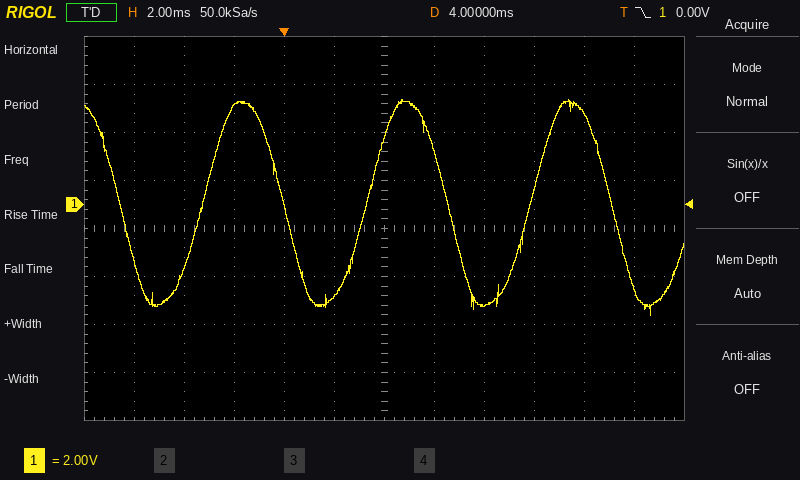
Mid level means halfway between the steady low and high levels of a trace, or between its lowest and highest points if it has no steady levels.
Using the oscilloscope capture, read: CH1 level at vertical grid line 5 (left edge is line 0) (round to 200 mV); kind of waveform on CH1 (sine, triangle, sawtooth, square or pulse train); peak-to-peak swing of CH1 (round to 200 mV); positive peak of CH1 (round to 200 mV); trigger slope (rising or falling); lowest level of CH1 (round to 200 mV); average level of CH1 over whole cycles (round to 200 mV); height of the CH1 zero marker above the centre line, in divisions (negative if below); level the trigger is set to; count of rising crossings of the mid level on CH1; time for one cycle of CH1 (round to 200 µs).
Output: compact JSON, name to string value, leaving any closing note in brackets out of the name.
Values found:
{"CH1 level at vertical grid line 5 (left edge is line 0)": "-3.8 V", "kind of waveform on CH1": "sine", "peak-to-peak swing of CH1": "9.0 V", "positive peak of CH1": "4.4 V", "trigger slope": "falling", "lowest level of CH1": "-4.6 V", "average level of CH1 over whole cycles": "0.0 V", "height of the CH1 zero marker above the centre line, in divisions": "+0.5 div", "level the trigger is set to": "0.00 V", "count of rising crossings of the mid level on CH1": "3", "time for one cycle of CH1": "6.6 ms"}
